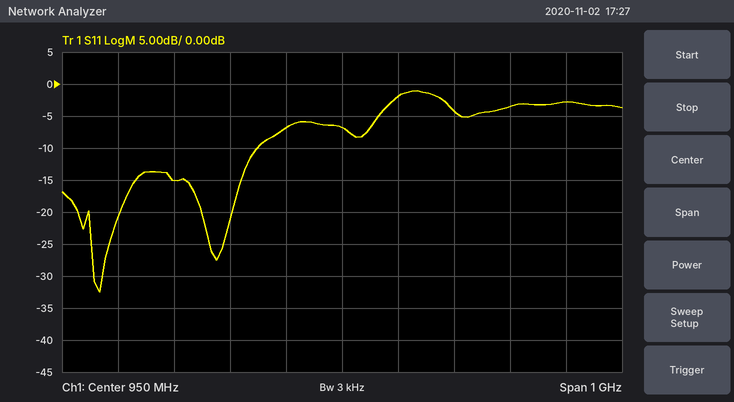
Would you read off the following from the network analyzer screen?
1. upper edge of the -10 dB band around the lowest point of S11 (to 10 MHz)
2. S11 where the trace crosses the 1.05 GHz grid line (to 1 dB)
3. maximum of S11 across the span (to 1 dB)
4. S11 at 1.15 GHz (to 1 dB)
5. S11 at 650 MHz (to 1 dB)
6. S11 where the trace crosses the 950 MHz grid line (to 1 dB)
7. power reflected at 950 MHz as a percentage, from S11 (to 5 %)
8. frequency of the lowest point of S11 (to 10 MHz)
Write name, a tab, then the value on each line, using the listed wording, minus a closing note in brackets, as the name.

upper edge of the -10 dB band around the lowest point of S11	800 MHz
S11 where the trace crosses the 1.05 GHz grid line	-2 dB
maximum of S11 across the span	-1 dB
S11 at 1.15 GHz	-4 dB
S11 at 650 MHz	-15 dB
S11 where the trace crosses the 950 MHz grid line	-7 dB
power reflected at 950 MHz as a percentage, from S11	20 %
frequency of the lowest point of S11	520 MHz
